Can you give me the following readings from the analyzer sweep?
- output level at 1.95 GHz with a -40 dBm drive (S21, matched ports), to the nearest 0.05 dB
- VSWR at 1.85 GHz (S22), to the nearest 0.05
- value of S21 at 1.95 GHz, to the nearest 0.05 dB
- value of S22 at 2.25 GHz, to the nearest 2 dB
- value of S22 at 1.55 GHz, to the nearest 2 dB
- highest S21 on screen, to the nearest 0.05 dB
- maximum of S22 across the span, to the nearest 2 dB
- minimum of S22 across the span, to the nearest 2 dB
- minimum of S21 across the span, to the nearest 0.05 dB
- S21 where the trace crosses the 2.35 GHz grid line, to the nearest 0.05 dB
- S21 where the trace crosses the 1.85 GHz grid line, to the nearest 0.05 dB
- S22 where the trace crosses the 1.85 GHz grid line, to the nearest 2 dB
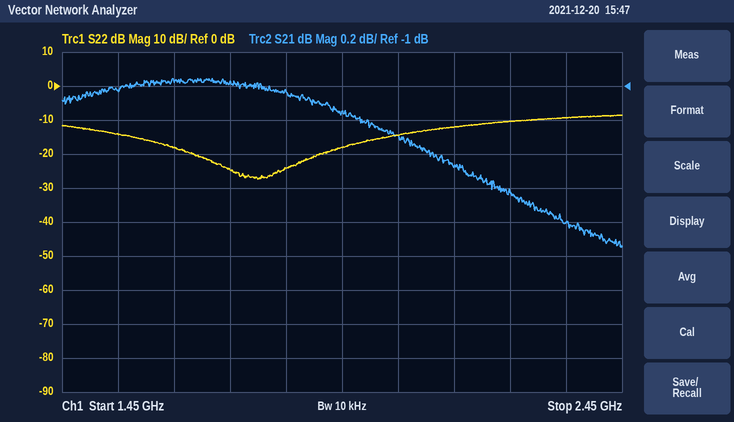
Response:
-41.15 dBm
1.15
-1.15 dB
-10 dB
-14 dB
-0.95 dB
-8 dB
-28 dB
-1.95 dB
-1.80 dB
-1.05 dB
-24 dB
